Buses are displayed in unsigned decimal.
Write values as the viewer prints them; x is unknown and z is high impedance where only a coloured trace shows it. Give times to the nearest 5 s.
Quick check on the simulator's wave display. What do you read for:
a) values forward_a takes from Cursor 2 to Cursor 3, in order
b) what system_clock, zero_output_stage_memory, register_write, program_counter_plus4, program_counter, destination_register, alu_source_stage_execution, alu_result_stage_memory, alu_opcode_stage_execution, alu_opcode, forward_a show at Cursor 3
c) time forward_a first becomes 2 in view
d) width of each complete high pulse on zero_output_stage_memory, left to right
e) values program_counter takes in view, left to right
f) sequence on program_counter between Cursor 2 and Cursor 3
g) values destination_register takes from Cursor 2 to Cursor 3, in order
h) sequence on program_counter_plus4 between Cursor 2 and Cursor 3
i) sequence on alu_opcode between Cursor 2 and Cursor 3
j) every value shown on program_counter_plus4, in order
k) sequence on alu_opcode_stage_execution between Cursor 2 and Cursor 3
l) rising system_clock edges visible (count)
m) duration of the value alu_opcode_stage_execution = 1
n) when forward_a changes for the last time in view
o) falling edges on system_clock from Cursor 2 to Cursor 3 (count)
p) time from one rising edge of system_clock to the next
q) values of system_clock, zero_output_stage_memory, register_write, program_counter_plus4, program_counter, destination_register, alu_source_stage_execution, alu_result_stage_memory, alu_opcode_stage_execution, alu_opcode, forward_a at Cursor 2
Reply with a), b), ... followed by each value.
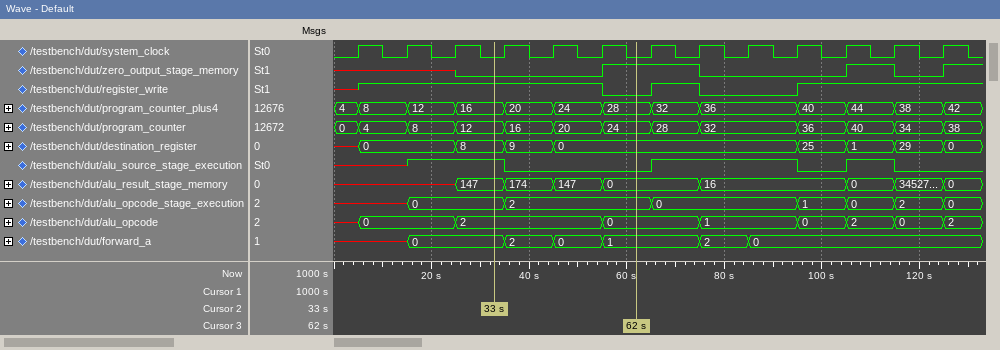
a) 0, 2, 0, 1
b) system_clock=0, zero_output_stage_memory=1, register_write=0, program_counter_plus4=28, program_counter=24, destination_register=0, alu_source_stage_execution=0, alu_result_stage_memory=0, alu_opcode_stage_execution=2, alu_opcode=0, forward_a=1
c) 35 s
d) 20 s, 10 s
e) 0, 4, 8, 12, 16, 20, 24, 28, 32, 36, 40, 34, 38
f) 12, 16, 20, 24
g) 8, 9, 0
h) 16, 20, 24, 28
i) 2, 0
j) 4, 8, 12, 16, 20, 24, 28, 32, 36, 40, 44, 38, 42
k) 0, 2
l) 13
m) 10 s
n) 85 s
o) 3
p) 10 s
q) system_clock=0, zero_output_stage_memory=0, register_write=1, program_counter_plus4=16, program_counter=12, destination_register=8, alu_source_stage_execution=1, alu_result_stage_memory=147, alu_opcode_stage_execution=0, alu_opcode=2, forward_a=0
